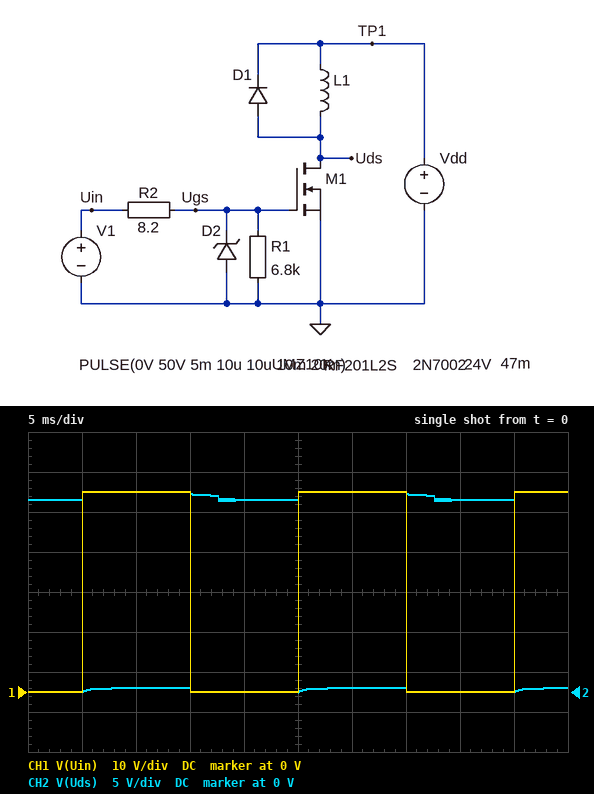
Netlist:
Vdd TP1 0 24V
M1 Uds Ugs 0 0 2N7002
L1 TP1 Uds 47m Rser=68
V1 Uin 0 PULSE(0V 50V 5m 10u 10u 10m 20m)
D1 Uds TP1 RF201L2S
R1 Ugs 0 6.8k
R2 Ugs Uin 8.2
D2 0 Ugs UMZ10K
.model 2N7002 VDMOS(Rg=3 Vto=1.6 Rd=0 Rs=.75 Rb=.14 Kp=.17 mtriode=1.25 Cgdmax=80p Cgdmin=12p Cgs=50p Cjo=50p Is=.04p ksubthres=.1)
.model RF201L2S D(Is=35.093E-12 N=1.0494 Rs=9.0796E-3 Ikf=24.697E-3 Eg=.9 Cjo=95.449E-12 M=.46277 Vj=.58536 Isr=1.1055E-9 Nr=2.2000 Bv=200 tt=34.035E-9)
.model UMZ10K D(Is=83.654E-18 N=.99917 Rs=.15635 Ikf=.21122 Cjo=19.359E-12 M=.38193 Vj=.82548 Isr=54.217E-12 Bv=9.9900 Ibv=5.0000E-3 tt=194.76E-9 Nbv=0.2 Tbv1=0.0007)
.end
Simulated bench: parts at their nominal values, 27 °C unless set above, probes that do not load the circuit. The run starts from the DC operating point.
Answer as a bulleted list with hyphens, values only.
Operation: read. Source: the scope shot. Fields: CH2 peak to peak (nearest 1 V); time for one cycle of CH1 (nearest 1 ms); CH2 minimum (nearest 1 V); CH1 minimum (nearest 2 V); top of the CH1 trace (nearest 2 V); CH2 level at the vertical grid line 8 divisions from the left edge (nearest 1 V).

- 25 V
- 20 ms
- 0 V
- 0 V
- 50 V
- 24 V
